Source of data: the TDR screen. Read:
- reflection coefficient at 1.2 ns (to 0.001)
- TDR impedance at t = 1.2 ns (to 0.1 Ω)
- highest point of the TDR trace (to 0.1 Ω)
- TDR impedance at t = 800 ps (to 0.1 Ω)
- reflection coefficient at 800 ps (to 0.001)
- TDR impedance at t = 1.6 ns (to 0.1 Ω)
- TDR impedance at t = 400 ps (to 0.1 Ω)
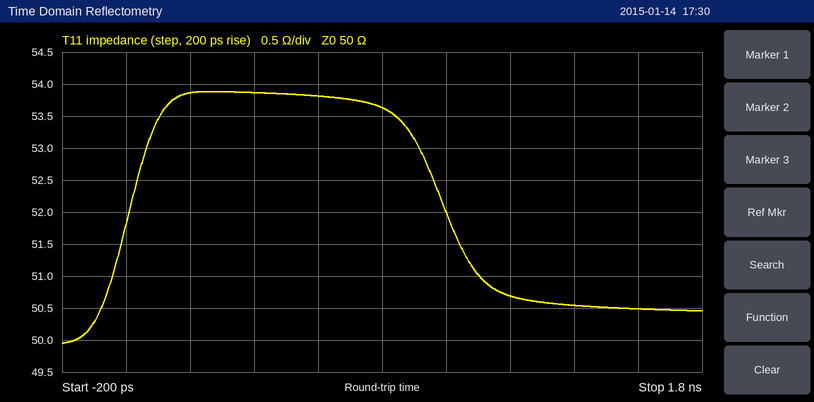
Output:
+0.007
50.7 Ω
53.9 Ω
53.6 Ω
+0.035
50.5 Ω
53.9 Ω
